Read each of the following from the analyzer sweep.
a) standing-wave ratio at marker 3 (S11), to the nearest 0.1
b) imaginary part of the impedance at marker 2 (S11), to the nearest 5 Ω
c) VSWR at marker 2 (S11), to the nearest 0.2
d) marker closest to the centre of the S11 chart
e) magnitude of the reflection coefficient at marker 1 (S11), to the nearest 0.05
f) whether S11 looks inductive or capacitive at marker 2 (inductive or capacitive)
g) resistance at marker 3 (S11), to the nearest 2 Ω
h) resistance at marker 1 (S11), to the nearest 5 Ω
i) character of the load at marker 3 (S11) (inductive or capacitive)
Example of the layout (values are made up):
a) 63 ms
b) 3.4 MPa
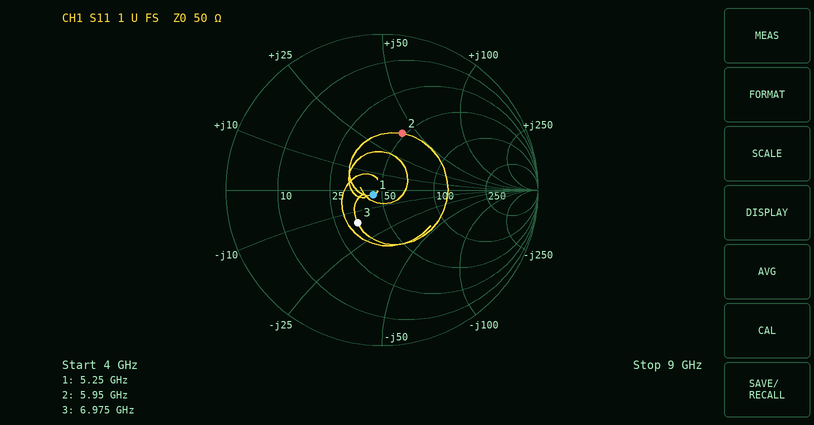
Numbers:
a) 1.7
b) +40 Ω
c) 2.2
d) marker 1
e) 0.05
f) inductive
g) 34 Ω
h) 45 Ω
i) capacitive
